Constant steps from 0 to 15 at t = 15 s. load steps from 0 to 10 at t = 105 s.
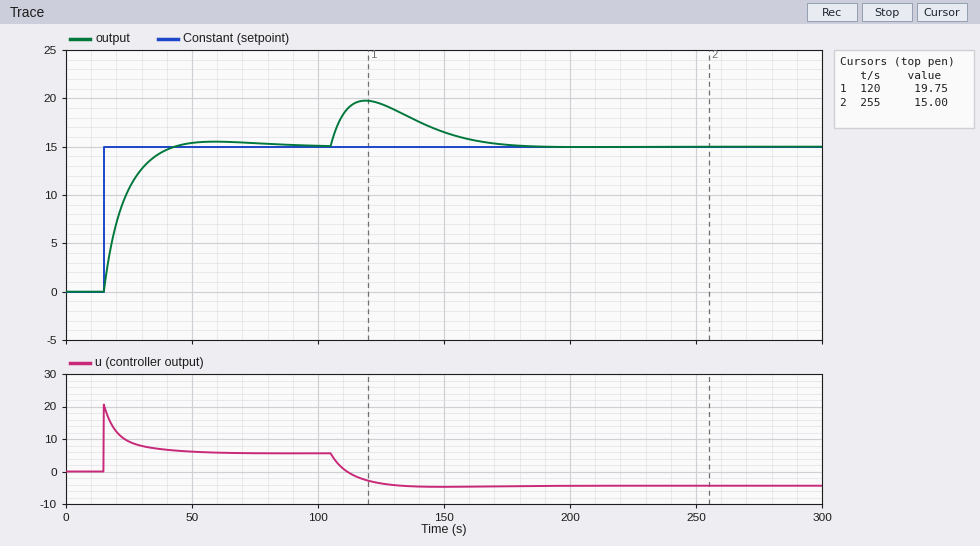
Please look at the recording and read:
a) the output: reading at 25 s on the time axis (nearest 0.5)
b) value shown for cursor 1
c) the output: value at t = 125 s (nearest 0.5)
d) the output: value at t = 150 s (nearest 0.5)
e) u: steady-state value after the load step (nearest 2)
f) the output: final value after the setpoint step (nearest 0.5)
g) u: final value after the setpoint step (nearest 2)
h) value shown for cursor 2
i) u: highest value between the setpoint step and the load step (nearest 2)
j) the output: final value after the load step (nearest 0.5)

10.5
19.75
19.5
16.5
-4
15.0
6
15.00
20
15.0
